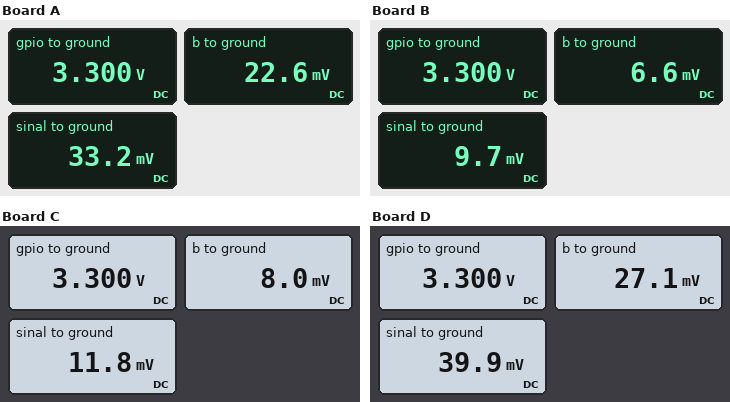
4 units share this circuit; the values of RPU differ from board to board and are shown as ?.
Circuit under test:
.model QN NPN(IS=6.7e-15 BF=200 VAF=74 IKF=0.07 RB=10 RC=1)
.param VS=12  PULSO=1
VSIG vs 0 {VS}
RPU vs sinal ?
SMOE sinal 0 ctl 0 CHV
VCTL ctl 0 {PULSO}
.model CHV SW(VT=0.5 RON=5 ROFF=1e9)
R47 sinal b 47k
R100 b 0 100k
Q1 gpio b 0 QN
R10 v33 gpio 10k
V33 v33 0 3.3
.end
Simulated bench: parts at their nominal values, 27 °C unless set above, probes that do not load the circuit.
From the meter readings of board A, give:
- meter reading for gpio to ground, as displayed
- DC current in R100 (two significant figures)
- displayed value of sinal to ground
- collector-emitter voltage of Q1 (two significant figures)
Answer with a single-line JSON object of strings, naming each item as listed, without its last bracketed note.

{"meter reading for gpio to ground, as displayed": "3.300 V", "DC current in R100": "230 nA", "displayed value of sinal to ground": "33.2 mV", "collector-emitter voltage of Q1": "3.3 V"}
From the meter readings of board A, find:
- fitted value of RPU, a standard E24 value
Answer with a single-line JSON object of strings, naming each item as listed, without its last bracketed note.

{"fitted value of RPU, a standard E24 value": "1.8 kΩ"}
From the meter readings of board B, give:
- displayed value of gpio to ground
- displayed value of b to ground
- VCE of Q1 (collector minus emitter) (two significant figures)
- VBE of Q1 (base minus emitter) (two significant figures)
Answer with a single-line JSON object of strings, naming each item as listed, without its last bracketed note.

{"displayed value of gpio to ground": "3.300 V", "displayed value of b to ground": "6.6 mV", "VCE of Q1 (collector minus emitter)": "3.3 V", "VBE of Q1 (base minus emitter)": "6.6 mV"}
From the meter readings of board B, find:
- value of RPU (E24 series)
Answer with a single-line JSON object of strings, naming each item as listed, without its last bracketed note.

{"value of RPU": "6.2 kΩ"}
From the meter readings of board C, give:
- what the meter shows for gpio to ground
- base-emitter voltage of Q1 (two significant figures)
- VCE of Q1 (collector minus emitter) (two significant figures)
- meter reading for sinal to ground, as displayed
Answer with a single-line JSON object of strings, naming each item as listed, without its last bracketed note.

{"what the meter shows for gpio to ground": "3.300 V", "base-emitter voltage of Q1": "8.0 mV", "VCE of Q1 (collector minus emitter)": "3.3 V", "meter reading for sinal to ground, as displayed": "11.8 mV"}
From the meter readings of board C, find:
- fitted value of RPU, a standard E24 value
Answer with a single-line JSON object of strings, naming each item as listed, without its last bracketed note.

{"fitted value of RPU, a standard E24 value": "5.1 kΩ"}
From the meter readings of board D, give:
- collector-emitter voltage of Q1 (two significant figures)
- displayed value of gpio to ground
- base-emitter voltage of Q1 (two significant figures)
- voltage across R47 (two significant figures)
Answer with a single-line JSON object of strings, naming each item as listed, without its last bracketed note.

{"collector-emitter voltage of Q1": "3.3 V", "displayed value of gpio to ground": "3.300 V", "base-emitter voltage of Q1": "27 mV", "voltage across R47": "13 mV"}
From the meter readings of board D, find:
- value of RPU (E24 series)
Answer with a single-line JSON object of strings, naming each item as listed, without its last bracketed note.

{"value of RPU": "1.5 kΩ"}
